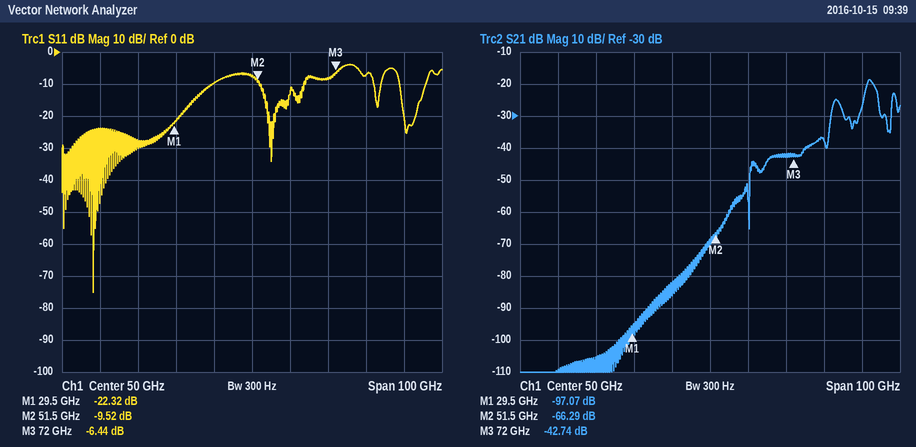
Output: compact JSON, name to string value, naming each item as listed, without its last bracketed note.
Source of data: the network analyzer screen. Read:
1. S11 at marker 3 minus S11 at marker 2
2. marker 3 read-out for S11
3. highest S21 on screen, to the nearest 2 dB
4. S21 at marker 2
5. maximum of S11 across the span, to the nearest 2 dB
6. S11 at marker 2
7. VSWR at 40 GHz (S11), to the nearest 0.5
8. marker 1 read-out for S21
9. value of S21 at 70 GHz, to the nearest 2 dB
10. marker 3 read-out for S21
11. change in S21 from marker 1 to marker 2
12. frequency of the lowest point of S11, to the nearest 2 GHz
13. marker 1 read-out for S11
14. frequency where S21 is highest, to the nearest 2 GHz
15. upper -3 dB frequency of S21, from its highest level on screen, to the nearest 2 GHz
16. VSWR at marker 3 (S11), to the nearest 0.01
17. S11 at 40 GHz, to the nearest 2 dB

{"S11 at marker 3 minus S11 at marker 2": "3.08 dB", "marker 3 read-out for S11": "-6.44 dB", "highest S21 on screen, to the nearest 2 dB": "-18 dB", "S21 at marker 2": "-66.29 dB", "maximum of S11 across the span, to the nearest 2 dB": "-4 dB", "S11 at marker 2": "-9.52 dB", "VSWR at 40 GHz (S11), to the nearest 0.5": "2.0", "marker 1 read-out for S21": "-97.07 dB", "value of S21 at 70 GHz, to the nearest 2 dB": "-42 dB", "marker 3 read-out for S21": "-42.74 dB", "change in S21 from marker 1 to marker 2": "30.78 dB", "frequency of the lowest point of S11, to the nearest 2 GHz": "8 GHz", "marker 1 read-out for S11": "-22.32 dB", "frequency where S21 is highest, to the nearest 2 GHz": "92 GHz", "upper -3 dB frequency of S21, from its highest level on screen, to the nearest 2 GHz": "94 GHz", "VSWR at marker 3 (S11), to the nearest 0.01": "2.82", "S11 at 40 GHz, to the nearest 2 dB": "-10 dB"}
